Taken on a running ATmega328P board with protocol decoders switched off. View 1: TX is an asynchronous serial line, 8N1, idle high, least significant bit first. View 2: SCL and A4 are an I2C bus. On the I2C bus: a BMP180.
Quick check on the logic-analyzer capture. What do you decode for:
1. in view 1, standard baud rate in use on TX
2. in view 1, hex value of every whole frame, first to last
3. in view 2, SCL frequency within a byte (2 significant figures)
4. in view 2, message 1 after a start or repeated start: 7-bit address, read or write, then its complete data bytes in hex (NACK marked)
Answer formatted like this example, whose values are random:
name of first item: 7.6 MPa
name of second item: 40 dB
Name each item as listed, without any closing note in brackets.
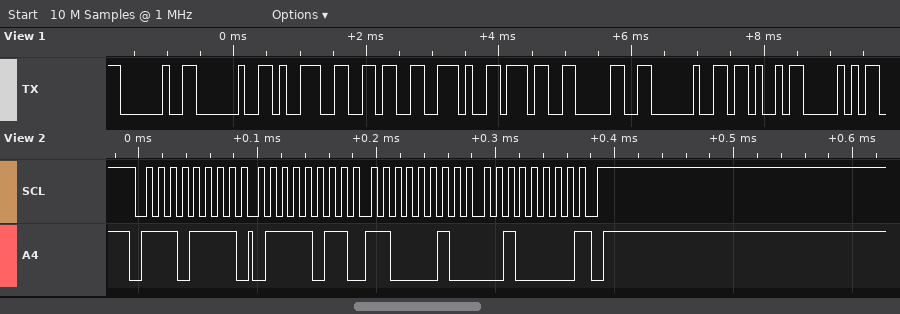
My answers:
in view 1, standard baud rate in use on TX: 9600 baud
in view 1, hex value of every whole frame, first to last: 20 20 39 36 2E 37 30 20 4B 50
in view 2, SCL frequency within a byte: 100 kHz
in view 2, message 1 after a start or repeated start: 7-bit address, read or write, then its complete data bytes in hex: 0x77 read: 7B C2 20 NACK
